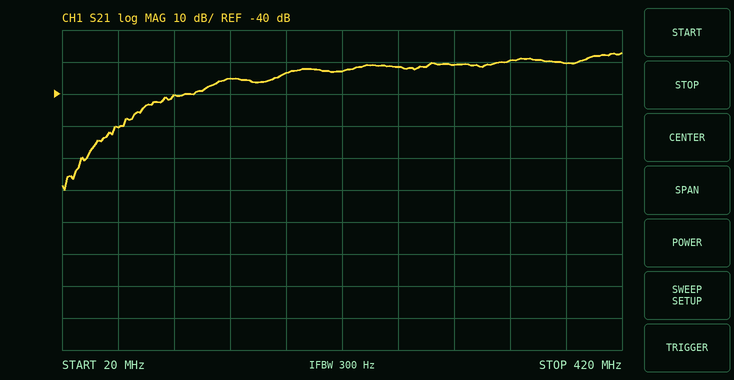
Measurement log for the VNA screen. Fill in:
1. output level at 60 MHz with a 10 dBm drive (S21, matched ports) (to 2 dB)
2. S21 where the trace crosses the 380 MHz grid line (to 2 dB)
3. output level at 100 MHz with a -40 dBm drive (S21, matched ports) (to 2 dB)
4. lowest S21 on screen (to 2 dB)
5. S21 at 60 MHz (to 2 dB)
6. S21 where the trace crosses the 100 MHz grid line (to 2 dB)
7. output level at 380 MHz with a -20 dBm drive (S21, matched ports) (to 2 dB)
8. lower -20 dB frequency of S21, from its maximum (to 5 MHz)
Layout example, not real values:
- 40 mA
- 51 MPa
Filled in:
- -40 dBm
- -30 dB
- -80 dBm
- -70 dB
- -50 dB
- -40 dB
- -50 dBm
- 70 MHz
